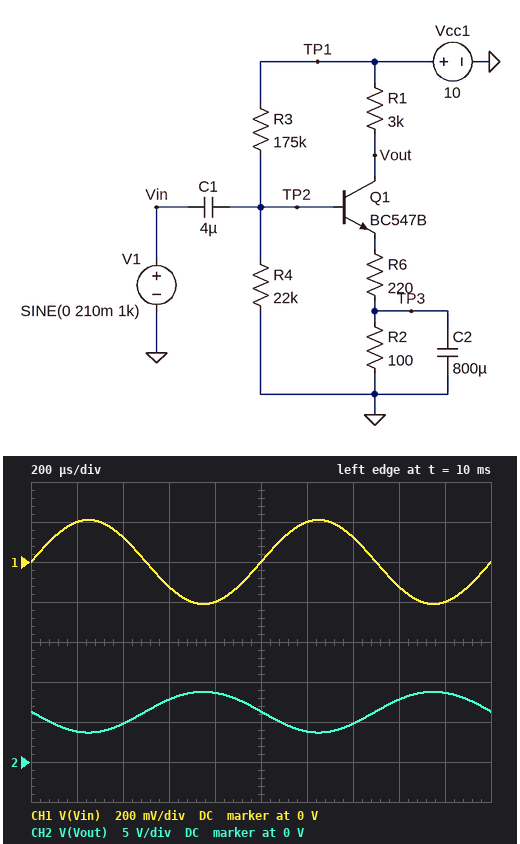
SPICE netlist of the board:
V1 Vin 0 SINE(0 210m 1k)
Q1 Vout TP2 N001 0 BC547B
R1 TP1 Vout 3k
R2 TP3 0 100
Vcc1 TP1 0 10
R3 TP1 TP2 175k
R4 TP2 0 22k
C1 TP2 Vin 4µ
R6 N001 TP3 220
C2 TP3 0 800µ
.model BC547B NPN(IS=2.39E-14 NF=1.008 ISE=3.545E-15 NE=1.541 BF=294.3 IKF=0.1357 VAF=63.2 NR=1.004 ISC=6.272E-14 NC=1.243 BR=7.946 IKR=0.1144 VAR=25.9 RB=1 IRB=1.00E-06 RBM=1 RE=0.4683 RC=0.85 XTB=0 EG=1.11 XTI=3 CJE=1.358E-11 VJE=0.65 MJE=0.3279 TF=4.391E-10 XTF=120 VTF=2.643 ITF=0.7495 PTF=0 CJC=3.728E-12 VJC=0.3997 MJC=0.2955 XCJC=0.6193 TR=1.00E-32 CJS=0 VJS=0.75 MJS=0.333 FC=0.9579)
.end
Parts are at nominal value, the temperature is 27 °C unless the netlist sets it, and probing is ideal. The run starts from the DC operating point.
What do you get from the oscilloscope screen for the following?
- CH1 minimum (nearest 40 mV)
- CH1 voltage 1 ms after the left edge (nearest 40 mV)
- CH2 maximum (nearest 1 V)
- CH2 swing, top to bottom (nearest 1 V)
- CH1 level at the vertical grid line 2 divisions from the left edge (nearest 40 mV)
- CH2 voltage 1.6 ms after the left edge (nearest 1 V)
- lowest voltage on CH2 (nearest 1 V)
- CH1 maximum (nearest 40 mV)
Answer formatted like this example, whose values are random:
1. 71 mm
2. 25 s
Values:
1. -200 mV
2. 0 V
3. 9 V
4. 5 V
5. 120 mV
6. 8 V
7. 4 V
8. 200 mV
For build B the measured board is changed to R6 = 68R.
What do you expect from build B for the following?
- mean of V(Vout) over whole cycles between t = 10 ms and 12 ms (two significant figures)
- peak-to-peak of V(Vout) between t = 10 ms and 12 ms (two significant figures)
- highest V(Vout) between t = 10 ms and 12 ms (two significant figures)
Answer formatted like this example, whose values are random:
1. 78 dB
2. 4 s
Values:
1. 6.1 V
2. 9.5 V
3. 10 V
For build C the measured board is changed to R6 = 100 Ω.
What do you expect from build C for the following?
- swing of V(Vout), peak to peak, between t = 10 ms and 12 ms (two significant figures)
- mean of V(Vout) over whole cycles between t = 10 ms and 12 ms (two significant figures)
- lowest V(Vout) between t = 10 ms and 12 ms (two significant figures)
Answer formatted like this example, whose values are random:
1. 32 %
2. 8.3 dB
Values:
1. 9.2 V
2. 5.4 V
3. 560 mV
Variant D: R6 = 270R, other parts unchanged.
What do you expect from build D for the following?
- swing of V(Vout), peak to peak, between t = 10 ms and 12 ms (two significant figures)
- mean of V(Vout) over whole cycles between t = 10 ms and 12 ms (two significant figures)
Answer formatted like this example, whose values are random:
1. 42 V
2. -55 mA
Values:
1. 4.2 V
2. 6.7 V
